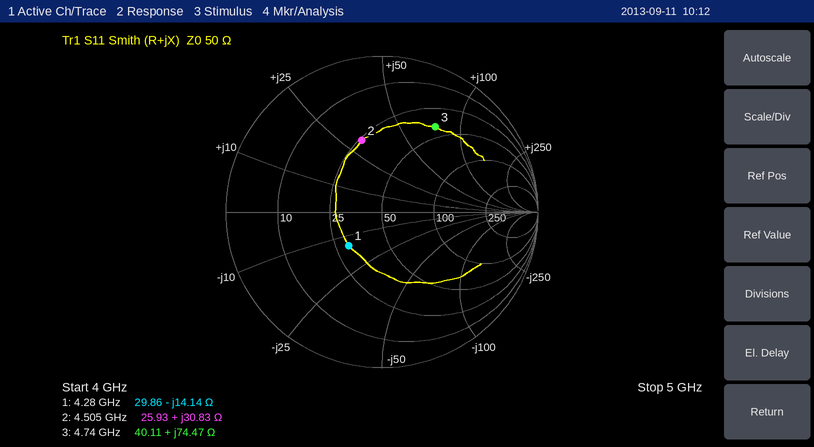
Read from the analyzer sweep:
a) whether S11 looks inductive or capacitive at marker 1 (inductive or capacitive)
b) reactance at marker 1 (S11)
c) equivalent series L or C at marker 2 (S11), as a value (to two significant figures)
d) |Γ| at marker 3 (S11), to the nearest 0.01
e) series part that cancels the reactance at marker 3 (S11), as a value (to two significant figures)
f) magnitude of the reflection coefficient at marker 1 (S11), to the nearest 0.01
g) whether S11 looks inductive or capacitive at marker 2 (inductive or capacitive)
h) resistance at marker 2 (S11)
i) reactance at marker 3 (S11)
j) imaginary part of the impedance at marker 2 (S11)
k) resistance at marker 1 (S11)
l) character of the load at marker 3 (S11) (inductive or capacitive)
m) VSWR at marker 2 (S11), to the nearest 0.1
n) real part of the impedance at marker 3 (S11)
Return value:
capacitive
-14.14 Ω
1.1 nH
0.64
450 fF
0.30
inductive
25.93 Ω
+74.47 Ω
+30.83 Ω
29.86 Ω
inductive
2.8
40.11 Ω
